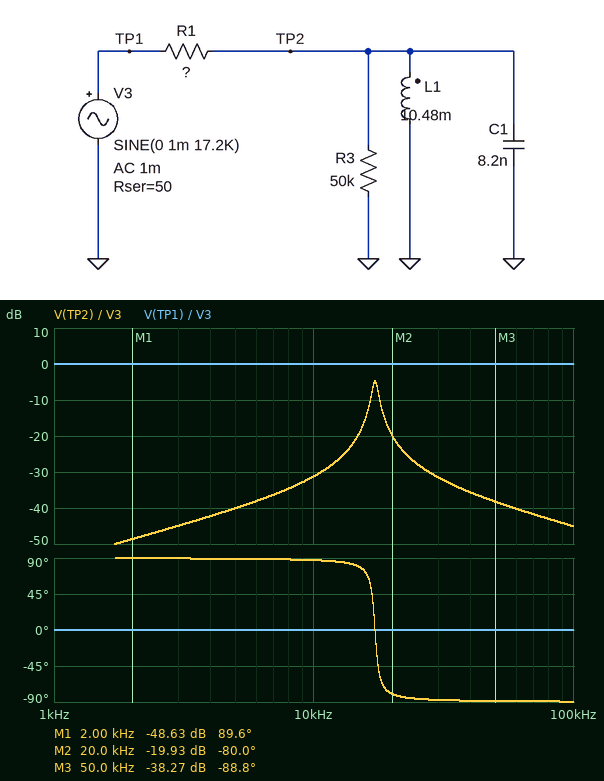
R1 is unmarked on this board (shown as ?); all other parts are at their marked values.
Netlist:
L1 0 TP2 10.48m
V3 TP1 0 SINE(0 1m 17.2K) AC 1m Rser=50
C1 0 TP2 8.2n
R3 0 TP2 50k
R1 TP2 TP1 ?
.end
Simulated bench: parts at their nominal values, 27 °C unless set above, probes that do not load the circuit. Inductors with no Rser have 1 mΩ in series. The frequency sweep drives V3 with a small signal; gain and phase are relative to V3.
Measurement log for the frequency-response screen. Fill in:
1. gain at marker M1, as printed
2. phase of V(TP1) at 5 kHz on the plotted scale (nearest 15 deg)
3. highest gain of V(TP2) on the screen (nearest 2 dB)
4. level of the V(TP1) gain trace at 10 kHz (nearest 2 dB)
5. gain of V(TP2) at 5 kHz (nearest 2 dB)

-48.63 dB
0 deg
-4 dB
0 dB
-40 dB
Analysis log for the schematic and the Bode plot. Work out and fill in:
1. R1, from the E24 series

36 kΩ
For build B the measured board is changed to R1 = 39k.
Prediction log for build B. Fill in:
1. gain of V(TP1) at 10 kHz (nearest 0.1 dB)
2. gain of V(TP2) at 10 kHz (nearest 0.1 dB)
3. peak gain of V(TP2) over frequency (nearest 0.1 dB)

0 dB
-31.9 dB
-5.0 dB
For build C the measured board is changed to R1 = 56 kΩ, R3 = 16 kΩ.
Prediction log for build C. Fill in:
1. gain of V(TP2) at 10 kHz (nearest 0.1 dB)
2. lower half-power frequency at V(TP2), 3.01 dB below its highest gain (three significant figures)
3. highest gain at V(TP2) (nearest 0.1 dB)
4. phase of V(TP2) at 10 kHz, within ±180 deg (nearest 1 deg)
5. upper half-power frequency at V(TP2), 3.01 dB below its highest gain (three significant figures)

-35.0 dB
16.4 kHz
-13.1 dB
85 deg
18.0 kHz
